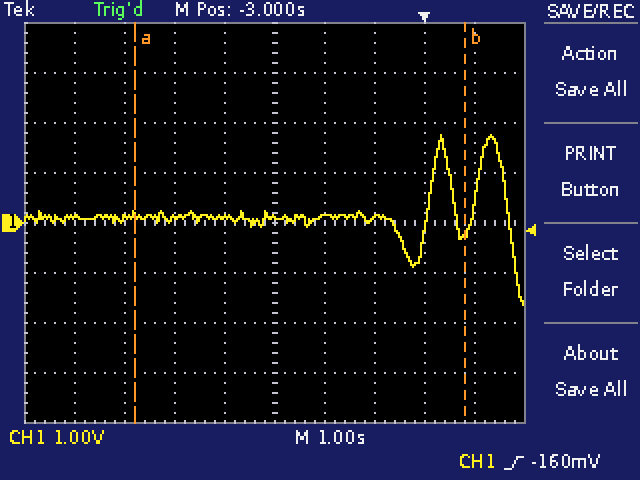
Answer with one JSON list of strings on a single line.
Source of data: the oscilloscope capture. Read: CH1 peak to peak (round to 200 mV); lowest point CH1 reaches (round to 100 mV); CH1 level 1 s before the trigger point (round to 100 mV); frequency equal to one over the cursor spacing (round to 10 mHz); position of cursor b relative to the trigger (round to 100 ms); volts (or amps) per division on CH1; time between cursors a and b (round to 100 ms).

["3.4 V", "-1.6 V", "100 mV", "150 mHz", "+800 ms", "1 V", "6.6 s"]
